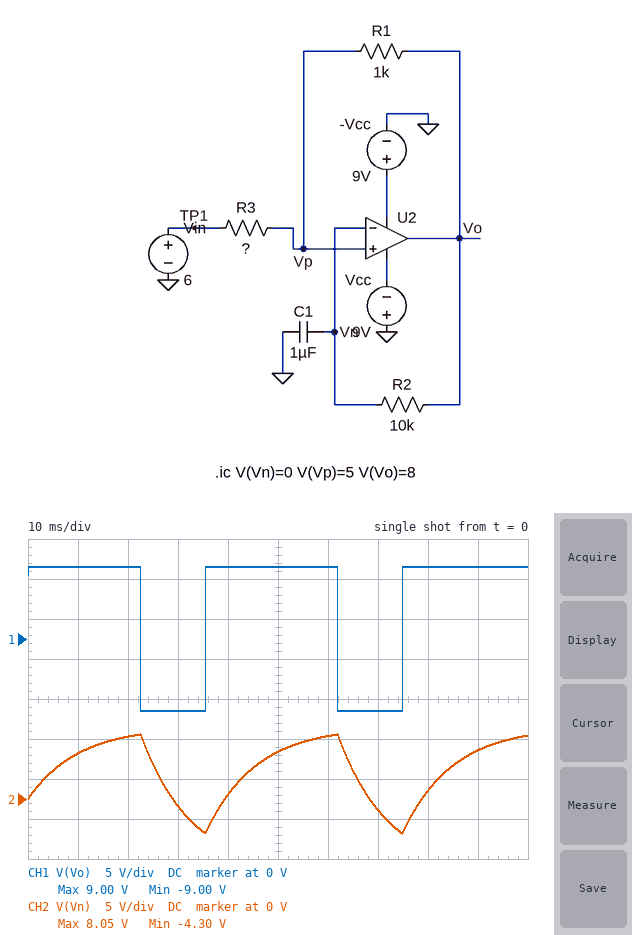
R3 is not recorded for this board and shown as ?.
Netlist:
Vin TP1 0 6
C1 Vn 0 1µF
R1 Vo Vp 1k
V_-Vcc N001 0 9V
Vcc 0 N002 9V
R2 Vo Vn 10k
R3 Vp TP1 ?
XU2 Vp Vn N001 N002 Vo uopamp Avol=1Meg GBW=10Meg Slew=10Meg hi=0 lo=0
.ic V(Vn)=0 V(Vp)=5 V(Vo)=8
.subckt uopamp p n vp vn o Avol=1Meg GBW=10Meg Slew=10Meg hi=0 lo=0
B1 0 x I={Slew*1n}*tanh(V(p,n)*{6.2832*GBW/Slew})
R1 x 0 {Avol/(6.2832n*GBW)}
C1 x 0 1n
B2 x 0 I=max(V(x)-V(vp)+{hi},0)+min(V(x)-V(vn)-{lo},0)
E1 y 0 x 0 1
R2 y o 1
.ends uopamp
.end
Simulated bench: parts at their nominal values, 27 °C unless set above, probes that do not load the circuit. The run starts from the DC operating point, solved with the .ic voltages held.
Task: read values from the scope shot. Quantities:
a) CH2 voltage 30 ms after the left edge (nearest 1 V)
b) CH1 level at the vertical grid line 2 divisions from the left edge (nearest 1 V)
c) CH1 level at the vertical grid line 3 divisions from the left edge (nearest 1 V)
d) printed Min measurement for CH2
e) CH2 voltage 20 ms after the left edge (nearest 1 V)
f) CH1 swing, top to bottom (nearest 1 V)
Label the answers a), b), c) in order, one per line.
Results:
a) -1 V
b) 9 V
c) -9 V
d) -4.30 V
e) 8 V
f) 18 V
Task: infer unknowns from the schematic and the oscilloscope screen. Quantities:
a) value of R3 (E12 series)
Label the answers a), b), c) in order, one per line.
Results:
a) 2.2 kΩ
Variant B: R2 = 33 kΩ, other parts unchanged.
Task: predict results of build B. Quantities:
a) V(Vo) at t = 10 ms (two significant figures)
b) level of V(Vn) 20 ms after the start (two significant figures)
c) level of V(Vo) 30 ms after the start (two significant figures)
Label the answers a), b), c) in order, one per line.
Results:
a) 9.0 V
b) 4.1 V
c) 9.0 V
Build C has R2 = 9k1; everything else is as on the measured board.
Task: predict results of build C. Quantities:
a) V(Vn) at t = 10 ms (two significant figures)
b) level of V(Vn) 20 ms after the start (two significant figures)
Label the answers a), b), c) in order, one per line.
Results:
a) 6.0 V
b) 8.0 V
